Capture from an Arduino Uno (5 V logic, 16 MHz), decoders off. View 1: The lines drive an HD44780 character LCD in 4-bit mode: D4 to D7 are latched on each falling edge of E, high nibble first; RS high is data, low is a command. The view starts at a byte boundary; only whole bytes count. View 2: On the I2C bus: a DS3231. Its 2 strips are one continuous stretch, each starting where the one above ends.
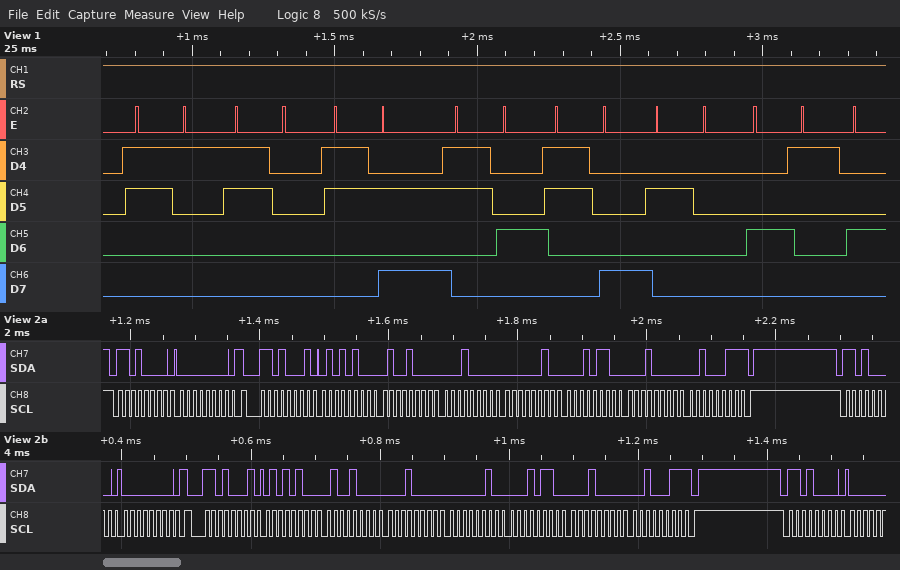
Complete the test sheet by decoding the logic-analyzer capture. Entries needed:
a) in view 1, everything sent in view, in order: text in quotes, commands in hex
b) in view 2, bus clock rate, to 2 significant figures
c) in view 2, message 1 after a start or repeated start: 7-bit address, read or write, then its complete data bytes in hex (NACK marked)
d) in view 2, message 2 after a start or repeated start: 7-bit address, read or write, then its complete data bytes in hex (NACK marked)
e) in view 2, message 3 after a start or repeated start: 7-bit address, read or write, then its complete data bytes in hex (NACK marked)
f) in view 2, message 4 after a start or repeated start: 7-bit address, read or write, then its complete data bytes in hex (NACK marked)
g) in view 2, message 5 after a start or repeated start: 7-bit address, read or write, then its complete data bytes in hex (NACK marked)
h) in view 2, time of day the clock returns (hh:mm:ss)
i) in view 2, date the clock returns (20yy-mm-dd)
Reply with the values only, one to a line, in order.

"10:48 A"
100 kHz
0x68 write: 00
0x68 read: 54 48 10 02 16 10 23 NACK
0x68 write: 00
0x68 read: 54 48 10 02 16 10 23 NACK
0x68 write
10:48:54
2023-10-16
